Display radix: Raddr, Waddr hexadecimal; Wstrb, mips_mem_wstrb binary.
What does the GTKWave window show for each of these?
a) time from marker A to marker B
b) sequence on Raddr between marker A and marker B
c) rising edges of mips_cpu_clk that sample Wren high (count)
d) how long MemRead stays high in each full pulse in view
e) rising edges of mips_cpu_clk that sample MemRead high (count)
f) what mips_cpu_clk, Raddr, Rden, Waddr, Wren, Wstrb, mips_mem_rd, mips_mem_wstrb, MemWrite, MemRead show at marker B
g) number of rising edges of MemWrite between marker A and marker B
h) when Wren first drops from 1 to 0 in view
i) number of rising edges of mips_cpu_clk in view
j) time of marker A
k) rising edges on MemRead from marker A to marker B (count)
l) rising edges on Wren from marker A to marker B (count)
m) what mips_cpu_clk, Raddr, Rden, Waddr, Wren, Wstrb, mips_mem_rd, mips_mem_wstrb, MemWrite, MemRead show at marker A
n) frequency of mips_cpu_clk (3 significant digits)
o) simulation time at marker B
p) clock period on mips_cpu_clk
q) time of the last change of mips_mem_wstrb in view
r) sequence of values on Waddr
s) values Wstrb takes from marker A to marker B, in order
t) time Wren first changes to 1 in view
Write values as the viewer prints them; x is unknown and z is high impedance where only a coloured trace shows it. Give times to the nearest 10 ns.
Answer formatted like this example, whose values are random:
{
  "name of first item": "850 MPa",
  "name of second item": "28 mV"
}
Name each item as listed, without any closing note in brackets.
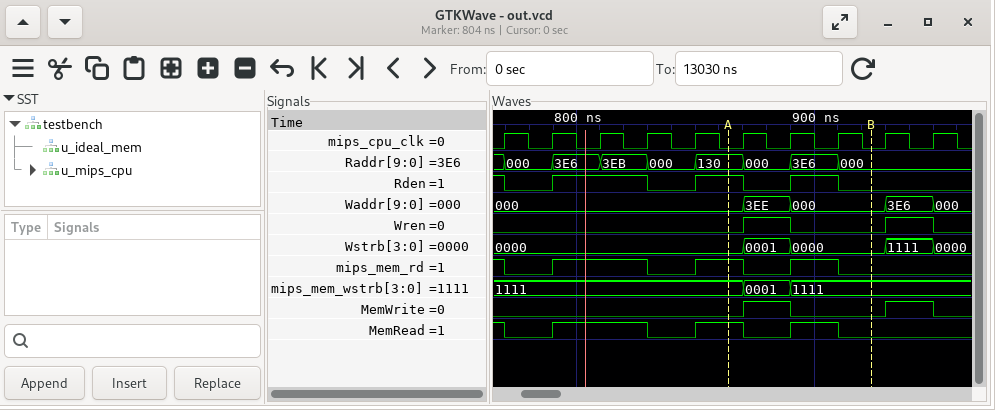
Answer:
{
  "time from marker A to marker B": "60 ns",
  "sequence on Raddr between marker A and marker B": "130, 000, 3E6, 000",
  "rising edges of mips_cpu_clk that sample Wren high": "2",
  "how long MemRead stays high in each full pulse in view": "40 ns, 20 ns, 20 ns",
  "rising edges of mips_cpu_clk that sample MemRead high": "5",
  "what mips_cpu_clk, Raddr, Rden, Waddr, Wren, Wstrb, mips_mem_rd, mips_mem_wstrb, MemWrite, MemRead show at marker B": "mips_cpu_clk=0, Raddr=000, Rden=0, Waddr=000, Wren=0, Wstrb=0000, mips_mem_rd=0, mips_mem_wstrb=1111, MemWrite=0, MemRead=0",
  "number of rising edges of MemWrite between marker A and marker B": "1",
  "when Wren first drops from 1 to 0 in view": "890 ns",
  "number of rising edges of mips_cpu_clk in view": "10",
  "time of marker A": "860 ns",
  "rising edges on MemRead from marker A to marker B": "1",
  "rising edges on Wren from marker A to marker B": "1",
  "what mips_cpu_clk, Raddr, Rden, Waddr, Wren, Wstrb, mips_mem_rd, mips_mem_wstrb, MemWrite, MemRead show at marker A": "mips_cpu_clk=0, Raddr=130, Rden=1, Waddr=000, Wren=0, Wstrb=0000, mips_mem_rd=1, mips_mem_wstrb=1111, MemWrite=0, MemRead=1",
  "frequency of mips_cpu_clk": "50.0 MHz",
  "simulation time at marker B": "920 ns",
  "clock period on mips_cpu_clk": "20 ns",
  "time of the last change of mips_mem_wstrb in view": "890 ns",
  "sequence of values on Waddr": "000, 3EE, 000, 3E6, 000",
  "values Wstrb takes from marker A to marker B, in order": "0000, 0001, 0000",
  "time Wren first changes to 1 in view": "870 ns"
}
